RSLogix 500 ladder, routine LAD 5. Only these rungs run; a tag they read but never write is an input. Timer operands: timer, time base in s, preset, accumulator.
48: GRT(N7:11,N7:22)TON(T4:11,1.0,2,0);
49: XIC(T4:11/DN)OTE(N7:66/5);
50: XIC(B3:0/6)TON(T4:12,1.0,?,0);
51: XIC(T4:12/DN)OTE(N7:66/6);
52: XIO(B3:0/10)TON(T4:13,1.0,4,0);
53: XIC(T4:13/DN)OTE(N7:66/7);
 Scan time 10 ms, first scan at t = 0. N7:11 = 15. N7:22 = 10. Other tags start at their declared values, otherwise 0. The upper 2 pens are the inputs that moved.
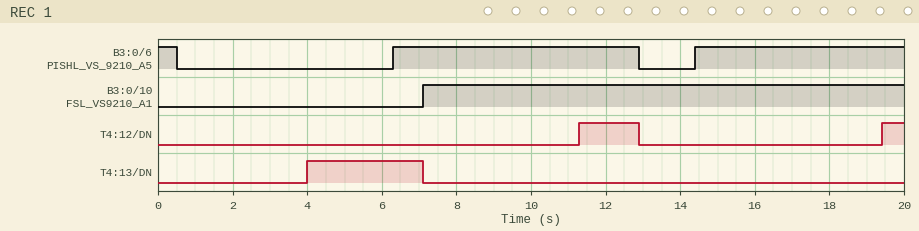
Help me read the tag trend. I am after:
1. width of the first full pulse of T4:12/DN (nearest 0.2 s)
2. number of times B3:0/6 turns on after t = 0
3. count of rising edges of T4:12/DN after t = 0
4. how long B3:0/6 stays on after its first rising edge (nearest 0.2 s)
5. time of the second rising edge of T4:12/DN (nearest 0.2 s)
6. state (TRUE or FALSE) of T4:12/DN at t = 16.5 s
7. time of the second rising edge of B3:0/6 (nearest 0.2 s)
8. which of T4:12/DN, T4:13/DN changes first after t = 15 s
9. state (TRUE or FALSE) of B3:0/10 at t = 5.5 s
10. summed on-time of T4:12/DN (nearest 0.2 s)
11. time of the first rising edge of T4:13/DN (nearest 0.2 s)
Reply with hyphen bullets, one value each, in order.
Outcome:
- 1.6 s
- 2
- 2
- 6.6 s
- 19.4 s
- FALSE
- 14.4 s
- T4:12/DN
- FALSE
- 2.2 s
- 4.0 s
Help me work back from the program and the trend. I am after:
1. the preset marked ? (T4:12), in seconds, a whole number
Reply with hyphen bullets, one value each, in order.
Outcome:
- 5 s
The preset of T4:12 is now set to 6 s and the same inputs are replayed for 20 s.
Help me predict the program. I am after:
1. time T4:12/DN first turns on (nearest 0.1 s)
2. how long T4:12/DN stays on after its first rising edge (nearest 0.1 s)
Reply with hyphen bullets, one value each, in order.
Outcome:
- 12.3 s
- 0.6 s
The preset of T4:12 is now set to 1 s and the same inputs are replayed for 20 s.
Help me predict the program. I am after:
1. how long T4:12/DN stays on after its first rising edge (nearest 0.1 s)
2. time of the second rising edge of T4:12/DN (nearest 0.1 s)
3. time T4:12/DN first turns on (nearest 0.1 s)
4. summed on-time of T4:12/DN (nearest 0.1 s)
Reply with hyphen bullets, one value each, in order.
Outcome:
- 5.6 s
- 15.4 s
- 7.3 s
- 10.2 s
